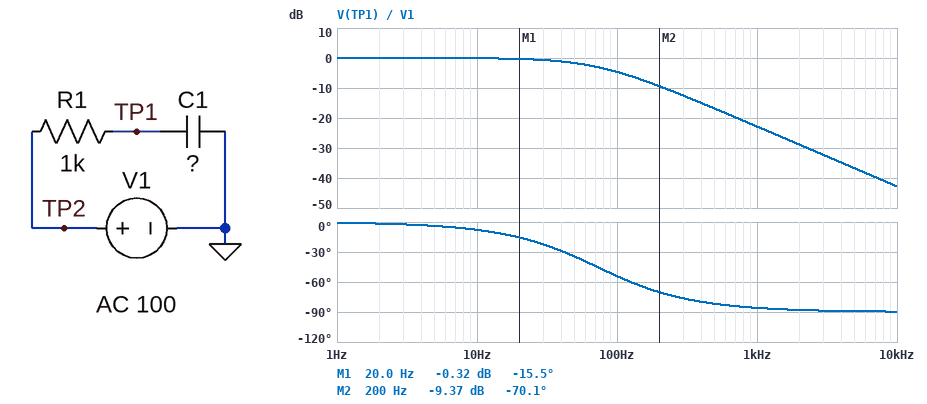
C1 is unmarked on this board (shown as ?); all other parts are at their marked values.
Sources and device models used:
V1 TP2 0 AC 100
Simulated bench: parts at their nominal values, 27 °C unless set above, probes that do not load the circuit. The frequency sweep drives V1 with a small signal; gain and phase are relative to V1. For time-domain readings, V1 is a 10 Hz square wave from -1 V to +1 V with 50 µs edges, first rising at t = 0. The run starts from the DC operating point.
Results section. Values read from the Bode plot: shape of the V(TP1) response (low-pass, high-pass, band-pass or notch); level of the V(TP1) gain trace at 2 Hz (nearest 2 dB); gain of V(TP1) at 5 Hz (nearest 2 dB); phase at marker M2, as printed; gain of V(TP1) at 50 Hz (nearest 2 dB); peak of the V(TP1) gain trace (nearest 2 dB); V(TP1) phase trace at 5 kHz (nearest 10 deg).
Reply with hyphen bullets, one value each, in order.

- low-pass
- 0 dB
- 0 dB
- -70.1 deg
- -2 dB
- 0 dB
- -90 deg
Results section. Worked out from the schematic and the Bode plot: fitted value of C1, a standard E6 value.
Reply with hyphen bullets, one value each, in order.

- 2.2 µF
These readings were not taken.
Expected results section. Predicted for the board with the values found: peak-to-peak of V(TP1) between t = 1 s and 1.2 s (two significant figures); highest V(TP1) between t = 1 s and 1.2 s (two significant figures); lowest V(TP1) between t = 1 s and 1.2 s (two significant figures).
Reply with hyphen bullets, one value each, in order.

- 2.0 V
- 1.0 V
- -1.0 V
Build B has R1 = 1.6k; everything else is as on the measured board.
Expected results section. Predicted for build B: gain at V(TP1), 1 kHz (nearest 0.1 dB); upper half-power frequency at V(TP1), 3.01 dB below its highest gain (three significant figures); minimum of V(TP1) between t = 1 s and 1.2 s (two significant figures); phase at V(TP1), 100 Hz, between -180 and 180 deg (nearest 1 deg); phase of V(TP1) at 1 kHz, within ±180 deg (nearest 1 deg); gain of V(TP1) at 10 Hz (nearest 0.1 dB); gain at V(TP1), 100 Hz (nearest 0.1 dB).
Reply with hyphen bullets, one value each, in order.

- -26.9 dB
- 45.2 Hz
- -1.0 V
- -66 deg
- -87 deg
- -0.2 dB
- -7.7 dB
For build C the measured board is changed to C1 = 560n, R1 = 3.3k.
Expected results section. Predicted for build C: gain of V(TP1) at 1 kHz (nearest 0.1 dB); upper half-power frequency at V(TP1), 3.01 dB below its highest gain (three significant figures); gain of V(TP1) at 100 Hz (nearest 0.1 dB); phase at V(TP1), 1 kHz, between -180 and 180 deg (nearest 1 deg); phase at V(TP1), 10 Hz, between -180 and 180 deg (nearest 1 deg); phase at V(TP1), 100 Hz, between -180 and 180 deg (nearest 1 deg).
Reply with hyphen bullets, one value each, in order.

- -21.3 dB
- 86.1 Hz
- -3.7 dB
- -85 deg
- -7 deg
- -49 deg
